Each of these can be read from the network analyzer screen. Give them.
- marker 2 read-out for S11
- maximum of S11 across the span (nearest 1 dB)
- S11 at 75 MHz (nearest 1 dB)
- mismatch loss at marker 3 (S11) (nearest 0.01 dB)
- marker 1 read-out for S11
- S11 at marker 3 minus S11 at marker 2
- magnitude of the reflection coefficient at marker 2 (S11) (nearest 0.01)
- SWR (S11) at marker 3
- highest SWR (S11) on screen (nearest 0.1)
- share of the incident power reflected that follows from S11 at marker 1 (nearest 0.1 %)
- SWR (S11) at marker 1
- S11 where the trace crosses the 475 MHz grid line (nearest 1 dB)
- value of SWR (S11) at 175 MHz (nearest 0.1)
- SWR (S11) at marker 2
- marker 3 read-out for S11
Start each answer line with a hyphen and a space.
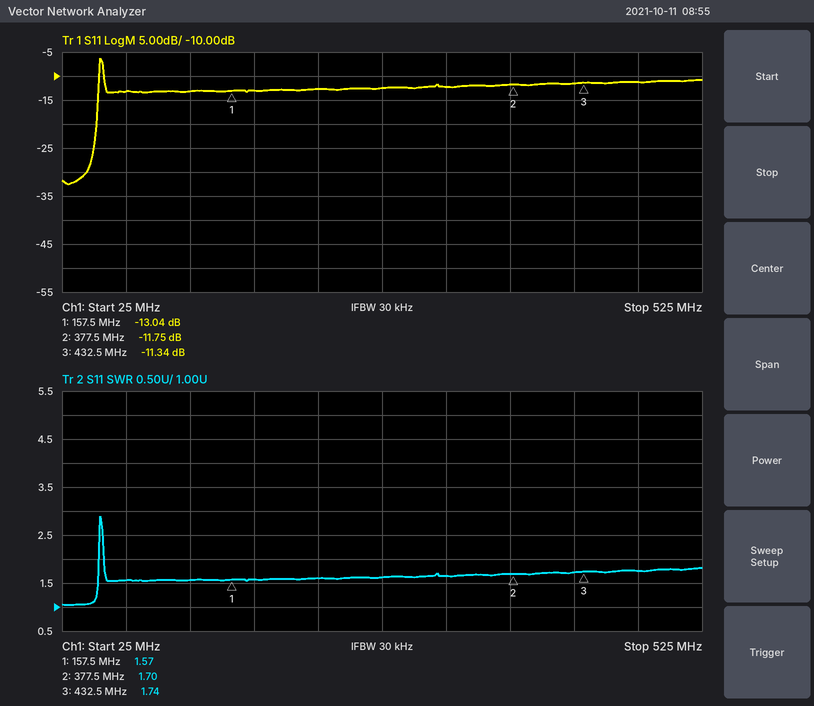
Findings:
- -11.75 dB
- -6 dB
- -13 dB
- 0.33 dB
- -13.04 dB
- 0.41 dB
- 0.26
- 1.74
- 2.9
- 5.0 %
- 1.57
- -11 dB
- 1.6
- 1.70
- -11.34 dB
